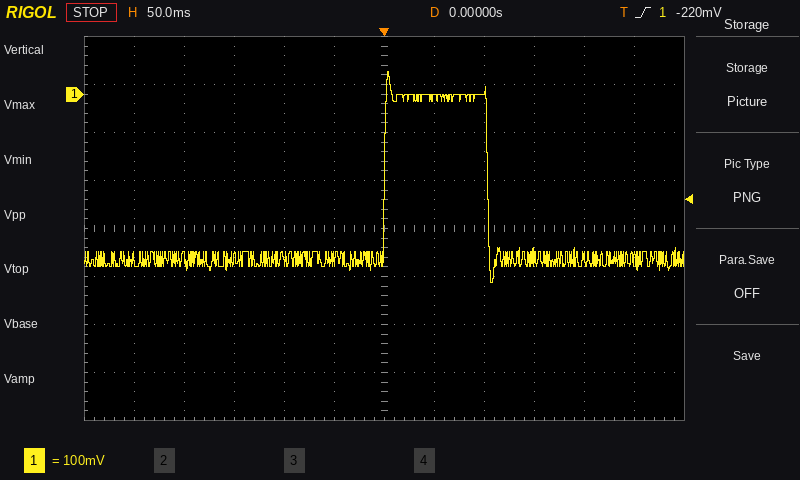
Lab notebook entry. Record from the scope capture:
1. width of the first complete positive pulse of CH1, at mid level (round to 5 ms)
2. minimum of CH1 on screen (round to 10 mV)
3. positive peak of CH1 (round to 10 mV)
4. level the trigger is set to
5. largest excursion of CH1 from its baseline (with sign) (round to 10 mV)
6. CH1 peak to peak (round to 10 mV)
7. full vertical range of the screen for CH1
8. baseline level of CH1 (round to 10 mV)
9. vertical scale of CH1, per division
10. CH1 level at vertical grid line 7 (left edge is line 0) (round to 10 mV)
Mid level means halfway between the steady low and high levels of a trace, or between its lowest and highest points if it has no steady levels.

105 ms
-390 mV
50 mV
-220 mV
+390 mV
440 mV
800 mV
-340 mV
100 mV
-10 mV
